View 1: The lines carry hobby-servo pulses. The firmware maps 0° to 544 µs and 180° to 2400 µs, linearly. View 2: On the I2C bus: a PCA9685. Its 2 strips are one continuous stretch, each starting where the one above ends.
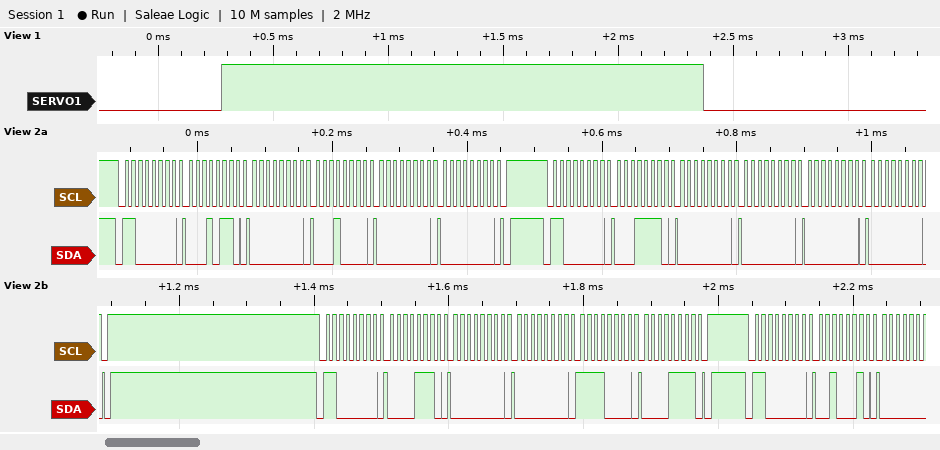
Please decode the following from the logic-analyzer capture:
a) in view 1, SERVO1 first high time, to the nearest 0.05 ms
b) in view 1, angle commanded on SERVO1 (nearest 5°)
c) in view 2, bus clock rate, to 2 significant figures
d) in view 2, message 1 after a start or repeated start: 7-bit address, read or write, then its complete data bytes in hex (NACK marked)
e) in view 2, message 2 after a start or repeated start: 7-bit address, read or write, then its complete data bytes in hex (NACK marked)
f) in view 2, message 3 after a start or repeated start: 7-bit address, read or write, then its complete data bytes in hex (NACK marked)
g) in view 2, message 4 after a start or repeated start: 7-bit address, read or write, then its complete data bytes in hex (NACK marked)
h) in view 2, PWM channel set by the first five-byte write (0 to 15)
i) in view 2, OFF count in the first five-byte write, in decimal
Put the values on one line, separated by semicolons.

2.10 ms; 150°; 100 kHz; 0x60 write: 16 00 10 00 00; 0x60 write: 1E 00 00 00 00; 0x60 write: 0E 00 00 F0 0F; 0x60 write: 22; 4; 0
